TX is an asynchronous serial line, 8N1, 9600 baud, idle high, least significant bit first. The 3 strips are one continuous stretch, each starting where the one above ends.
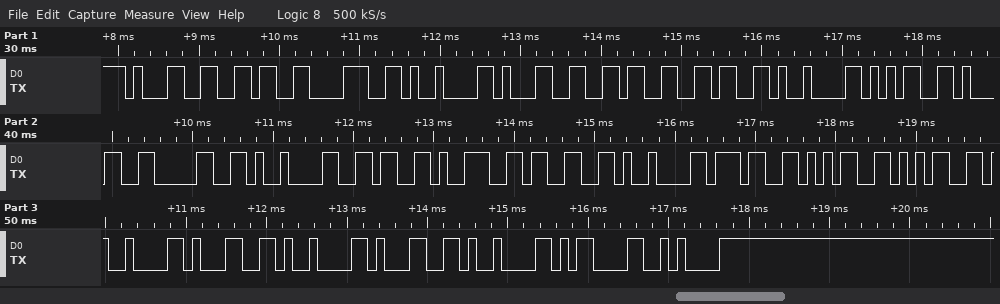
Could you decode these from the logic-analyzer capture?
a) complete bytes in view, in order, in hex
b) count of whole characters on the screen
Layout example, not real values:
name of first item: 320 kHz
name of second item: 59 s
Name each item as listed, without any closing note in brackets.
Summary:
complete bytes in view, in order, in hex: 0x31 0x36 0x38 0x09 0x31 0x36 0x36 0x09 0x35 0x31 0x30 0x09 0x36 0x39 0x33 0x09 0x37 0x35 0x35 0x09 0x31 0x09 0x31 0x09 0x0D 0x0A
count of whole characters on the screen: 26
